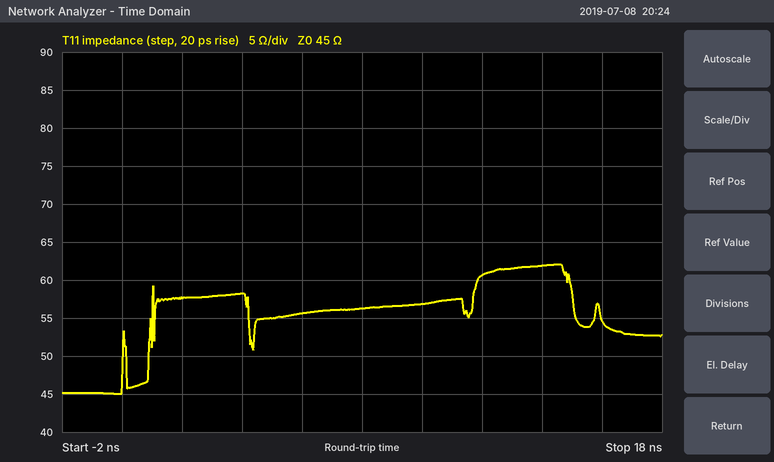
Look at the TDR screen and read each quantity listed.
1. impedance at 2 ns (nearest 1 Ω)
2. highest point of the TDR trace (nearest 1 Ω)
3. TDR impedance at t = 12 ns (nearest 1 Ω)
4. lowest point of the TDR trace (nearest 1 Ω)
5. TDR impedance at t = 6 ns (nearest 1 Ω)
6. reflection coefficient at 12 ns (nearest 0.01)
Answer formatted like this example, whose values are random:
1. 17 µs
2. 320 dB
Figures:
1. 58 Ω
2. 62 Ω
3. 61 Ω
4. 45 Ω
5. 56 Ω
6. +0.15
